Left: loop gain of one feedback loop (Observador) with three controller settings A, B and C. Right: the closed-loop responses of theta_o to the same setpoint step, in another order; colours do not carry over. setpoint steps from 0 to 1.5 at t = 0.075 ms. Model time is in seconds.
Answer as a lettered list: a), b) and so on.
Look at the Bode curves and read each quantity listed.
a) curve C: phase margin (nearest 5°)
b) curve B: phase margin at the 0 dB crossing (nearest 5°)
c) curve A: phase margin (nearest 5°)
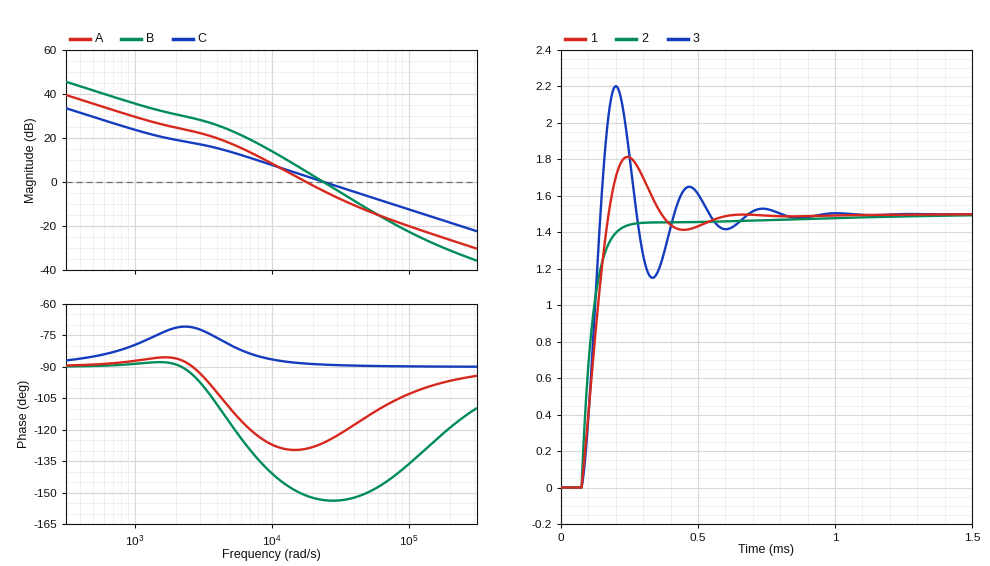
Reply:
a) 90°
b) 25°
c) 50°
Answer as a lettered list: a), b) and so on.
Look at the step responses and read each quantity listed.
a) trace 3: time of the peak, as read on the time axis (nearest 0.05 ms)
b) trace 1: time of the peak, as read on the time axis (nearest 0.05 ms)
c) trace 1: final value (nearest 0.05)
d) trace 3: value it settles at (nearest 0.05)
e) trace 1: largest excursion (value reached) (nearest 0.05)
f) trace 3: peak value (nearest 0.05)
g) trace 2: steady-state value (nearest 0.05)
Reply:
a) 0.20 ms
b) 0.25 ms
c) 1.50
d) 1.50
e) 1.80
f) 2.20
g) 1.50
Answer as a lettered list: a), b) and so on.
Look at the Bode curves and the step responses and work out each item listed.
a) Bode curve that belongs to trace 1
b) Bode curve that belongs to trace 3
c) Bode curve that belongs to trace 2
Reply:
a) A
b) B
c) C
